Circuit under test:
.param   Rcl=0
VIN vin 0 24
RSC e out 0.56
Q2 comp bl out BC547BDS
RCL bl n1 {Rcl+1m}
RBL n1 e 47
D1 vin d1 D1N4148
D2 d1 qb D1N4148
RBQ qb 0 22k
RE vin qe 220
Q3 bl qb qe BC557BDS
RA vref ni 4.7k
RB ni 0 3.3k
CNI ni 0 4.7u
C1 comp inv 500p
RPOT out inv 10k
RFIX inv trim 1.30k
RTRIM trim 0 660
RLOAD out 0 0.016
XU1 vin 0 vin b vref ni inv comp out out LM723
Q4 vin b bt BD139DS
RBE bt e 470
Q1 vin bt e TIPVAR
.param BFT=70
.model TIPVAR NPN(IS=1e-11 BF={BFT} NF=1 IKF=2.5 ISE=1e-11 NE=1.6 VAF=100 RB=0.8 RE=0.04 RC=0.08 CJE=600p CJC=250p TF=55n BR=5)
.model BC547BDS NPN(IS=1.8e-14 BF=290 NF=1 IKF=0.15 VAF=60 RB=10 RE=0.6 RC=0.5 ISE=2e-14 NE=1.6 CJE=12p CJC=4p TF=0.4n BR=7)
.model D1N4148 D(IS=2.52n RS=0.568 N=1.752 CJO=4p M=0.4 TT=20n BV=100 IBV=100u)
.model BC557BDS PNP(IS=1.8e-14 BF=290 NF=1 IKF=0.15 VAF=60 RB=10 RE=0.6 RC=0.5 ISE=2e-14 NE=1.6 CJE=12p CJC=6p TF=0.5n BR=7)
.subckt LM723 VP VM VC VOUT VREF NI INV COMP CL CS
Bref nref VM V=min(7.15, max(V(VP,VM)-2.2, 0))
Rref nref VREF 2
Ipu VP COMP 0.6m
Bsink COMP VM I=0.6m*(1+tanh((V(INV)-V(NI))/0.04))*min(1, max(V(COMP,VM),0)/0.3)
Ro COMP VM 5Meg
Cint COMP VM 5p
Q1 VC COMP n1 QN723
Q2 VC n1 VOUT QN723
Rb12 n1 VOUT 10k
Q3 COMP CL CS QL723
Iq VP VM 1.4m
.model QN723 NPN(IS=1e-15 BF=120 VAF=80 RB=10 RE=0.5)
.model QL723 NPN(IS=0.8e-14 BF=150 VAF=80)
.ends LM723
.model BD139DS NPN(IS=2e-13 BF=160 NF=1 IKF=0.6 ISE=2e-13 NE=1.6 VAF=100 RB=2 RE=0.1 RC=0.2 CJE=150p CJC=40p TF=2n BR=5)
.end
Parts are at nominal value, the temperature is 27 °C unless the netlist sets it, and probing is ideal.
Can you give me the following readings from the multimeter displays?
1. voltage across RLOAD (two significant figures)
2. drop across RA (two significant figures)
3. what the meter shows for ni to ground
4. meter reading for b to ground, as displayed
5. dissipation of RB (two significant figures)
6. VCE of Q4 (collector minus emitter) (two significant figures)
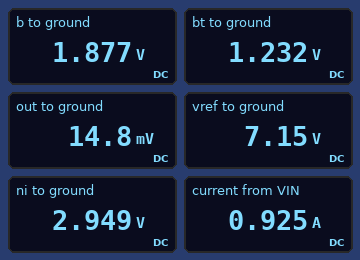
15 mV
4.2 V
2.949 V
1.877 V
2.6 mW
23 V
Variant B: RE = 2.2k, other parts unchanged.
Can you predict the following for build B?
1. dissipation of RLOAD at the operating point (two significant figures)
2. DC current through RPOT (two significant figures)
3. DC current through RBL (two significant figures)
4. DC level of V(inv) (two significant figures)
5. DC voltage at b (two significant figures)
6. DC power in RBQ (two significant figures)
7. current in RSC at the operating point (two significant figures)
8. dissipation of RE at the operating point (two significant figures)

19 mW
1.5 µA
260 µA
2.9 mV
2.0 V
24 mW
1.1 A
150 µW
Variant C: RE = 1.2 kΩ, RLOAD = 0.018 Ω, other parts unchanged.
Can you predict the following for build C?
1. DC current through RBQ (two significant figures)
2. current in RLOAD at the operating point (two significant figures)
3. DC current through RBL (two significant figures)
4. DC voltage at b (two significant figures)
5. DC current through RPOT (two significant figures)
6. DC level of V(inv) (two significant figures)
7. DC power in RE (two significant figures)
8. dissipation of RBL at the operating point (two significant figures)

1.0 mA
1.1 A
460 µA
2.0 V
1.6 µA
3.2 mV
260 µW
10 µW
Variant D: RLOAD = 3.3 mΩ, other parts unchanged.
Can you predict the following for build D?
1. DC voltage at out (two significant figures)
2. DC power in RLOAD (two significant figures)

3.0 mV
2.8 mW
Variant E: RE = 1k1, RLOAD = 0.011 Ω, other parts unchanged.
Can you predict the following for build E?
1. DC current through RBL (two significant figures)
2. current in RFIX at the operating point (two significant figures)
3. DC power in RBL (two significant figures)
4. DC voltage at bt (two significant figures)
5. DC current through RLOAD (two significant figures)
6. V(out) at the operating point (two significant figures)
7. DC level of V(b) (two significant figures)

500 µA
990 nA
12 µW
1.3 V
1.1 A
12 mV
2.0 V
